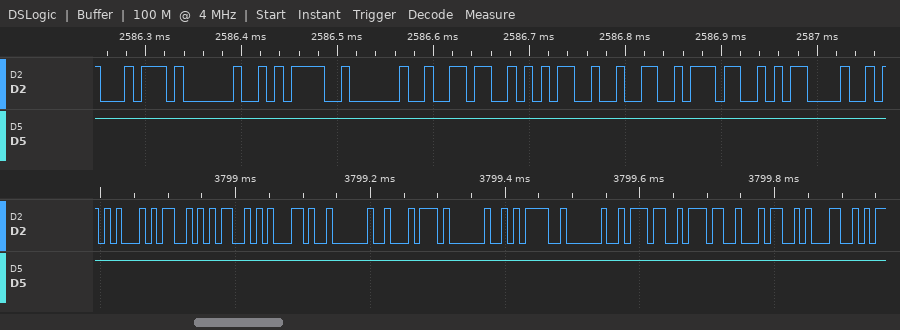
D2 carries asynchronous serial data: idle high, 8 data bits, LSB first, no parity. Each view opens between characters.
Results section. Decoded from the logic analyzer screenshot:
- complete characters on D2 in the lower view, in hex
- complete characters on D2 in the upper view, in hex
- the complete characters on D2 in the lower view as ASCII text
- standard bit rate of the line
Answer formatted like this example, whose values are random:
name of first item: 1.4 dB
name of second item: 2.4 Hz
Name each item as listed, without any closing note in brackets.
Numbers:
complete characters on D2 in the lower view, in hex: 45, 53, 53, 2C, 20, 74, 20, 3D, 20, 37, 37, 34, 31
complete characters on D2 in the upper view, in hex: 74, 20, 3D, 20, 36, 35, 32, 37, 0D
the complete characters on D2 in the lower view as ASCII text: "ESS, t = 7741"
standard bit rate of the line: 115200 baud
